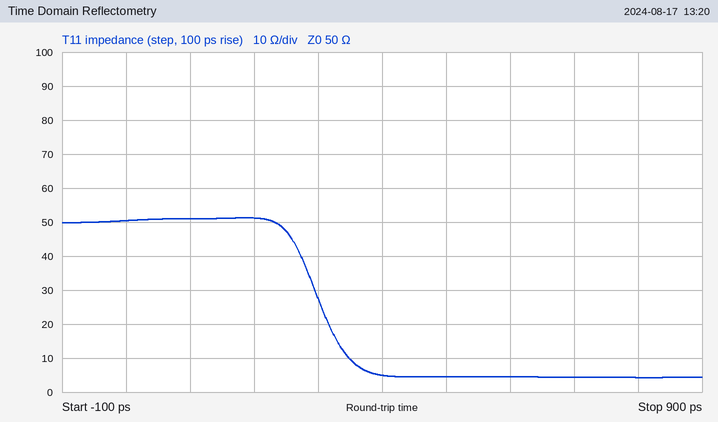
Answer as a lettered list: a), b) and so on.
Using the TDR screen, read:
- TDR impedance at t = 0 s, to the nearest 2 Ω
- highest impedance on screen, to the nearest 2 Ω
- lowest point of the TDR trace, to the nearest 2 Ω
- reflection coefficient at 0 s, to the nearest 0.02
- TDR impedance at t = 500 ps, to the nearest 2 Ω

a) 50 Ω
b) 52 Ω
c) 4 Ω
d) 0.00
e) 4 Ω
